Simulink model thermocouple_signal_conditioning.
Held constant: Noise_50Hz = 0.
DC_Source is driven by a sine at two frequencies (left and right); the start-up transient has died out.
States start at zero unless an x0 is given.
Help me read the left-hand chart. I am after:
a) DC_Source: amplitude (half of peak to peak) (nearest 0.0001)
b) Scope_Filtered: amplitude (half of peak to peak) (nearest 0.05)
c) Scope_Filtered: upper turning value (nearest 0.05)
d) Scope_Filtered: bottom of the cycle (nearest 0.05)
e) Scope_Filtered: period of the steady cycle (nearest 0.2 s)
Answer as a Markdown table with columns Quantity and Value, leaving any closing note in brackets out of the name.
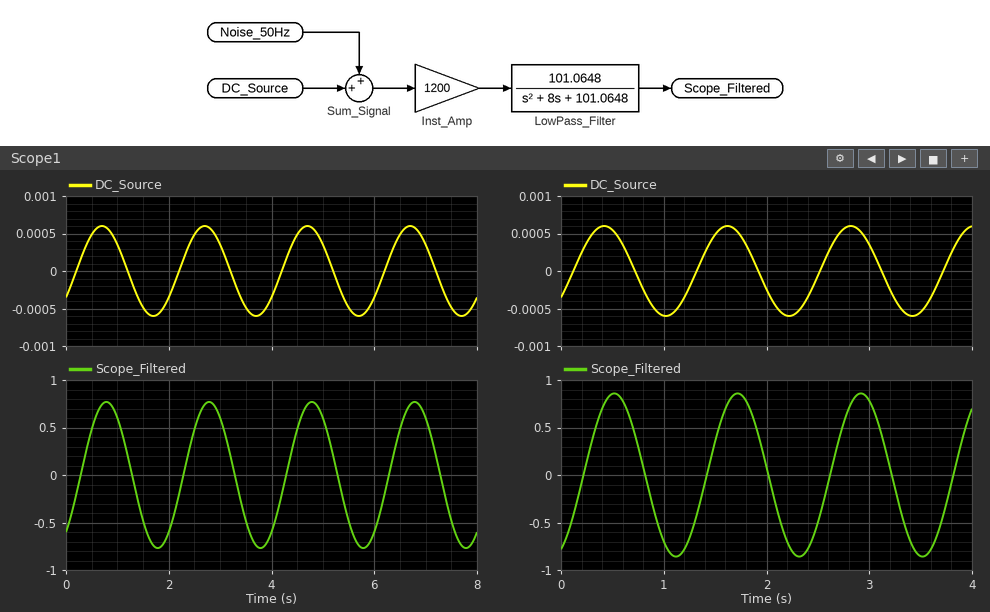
| Quantity | Value |
|---|---|
| DC_Source: amplitude (half of peak to peak) | 0.0006 |
| Scope_Filtered: amplitude (half of peak to peak) | 0.75 |
| Scope_Filtered: upper turning value | 0.75 |
| Scope_Filtered: bottom of the cycle | -0.75 |
| Scope_Filtered: period of the steady cycle | 2.0 s |
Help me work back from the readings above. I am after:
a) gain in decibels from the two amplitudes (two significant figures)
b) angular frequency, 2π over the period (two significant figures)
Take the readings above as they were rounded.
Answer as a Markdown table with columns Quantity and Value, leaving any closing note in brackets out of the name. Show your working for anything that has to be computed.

| Quantity | Value |
|---|---|
| gain in decibels from the two amplitudes | 20 log10(0.75 / 0.0006) = 62 dB |
| angular frequency, 2π over the period | 2π / 2 = 3.1 rad/s |
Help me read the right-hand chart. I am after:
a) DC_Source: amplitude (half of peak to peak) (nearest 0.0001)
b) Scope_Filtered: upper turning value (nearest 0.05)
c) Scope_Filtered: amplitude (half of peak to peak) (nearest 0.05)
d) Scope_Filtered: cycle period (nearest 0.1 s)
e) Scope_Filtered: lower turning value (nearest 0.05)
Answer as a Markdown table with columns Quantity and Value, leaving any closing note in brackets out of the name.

| Quantity | Value |
|---|---|
| DC_Source: amplitude (half of peak to peak) | 0.0006 |
| Scope_Filtered: upper turning value | 0.85 |
| Scope_Filtered: amplitude (half of peak to peak) | 0.85 |
| Scope_Filtered: cycle period | 1.2 s |
| Scope_Filtered: lower turning value | -0.85 |
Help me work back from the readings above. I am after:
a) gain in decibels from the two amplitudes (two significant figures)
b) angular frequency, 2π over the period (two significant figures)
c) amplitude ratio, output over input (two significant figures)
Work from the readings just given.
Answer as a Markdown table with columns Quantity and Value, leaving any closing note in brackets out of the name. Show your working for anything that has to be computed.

| Quantity | Value |
|---|---|
| gain in decibels from the two amplitudes | 20 log10(0.85 / 0.0006) = 63 dB |
| angular frequency, 2π over the period | 2π / 1.2 = 5.2 rad/s |
| amplitude ratio, output over input | 0.85 / 0.0006 = 1400 |
